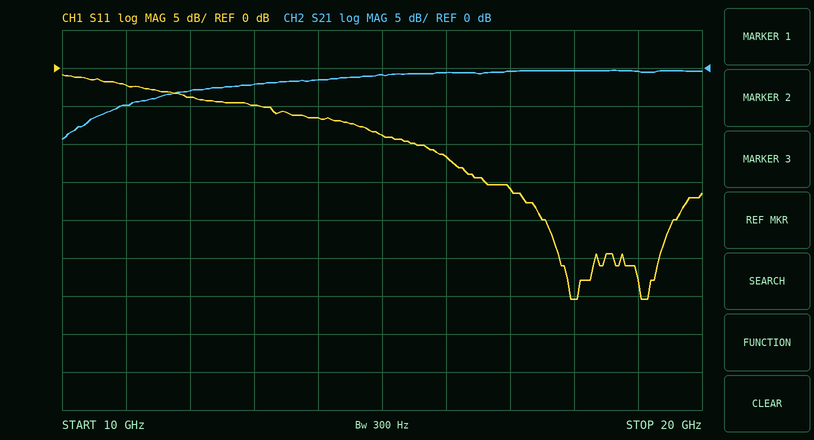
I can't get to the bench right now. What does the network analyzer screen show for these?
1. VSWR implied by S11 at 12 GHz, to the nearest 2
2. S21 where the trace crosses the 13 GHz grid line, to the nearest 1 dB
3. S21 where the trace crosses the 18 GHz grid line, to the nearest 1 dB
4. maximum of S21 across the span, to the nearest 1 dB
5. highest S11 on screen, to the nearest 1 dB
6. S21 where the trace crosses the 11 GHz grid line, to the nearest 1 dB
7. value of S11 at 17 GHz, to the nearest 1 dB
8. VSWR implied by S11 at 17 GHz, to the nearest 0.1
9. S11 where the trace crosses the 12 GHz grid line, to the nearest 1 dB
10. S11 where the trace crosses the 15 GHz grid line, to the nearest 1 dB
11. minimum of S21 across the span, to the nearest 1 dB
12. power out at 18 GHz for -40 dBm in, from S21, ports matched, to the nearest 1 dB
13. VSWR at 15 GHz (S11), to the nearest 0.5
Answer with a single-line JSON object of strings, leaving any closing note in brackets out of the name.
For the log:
{"VSWR implied by S11 at 12 GHz, to the nearest 2": "4", "S21 where the trace crosses the 13 GHz grid line, to the nearest 1 dB": "-2 dB", "S21 where the trace crosses the 18 GHz grid line, to the nearest 1 dB": "0 dB", "maximum of S21 across the span, to the nearest 1 dB": "0 dB", "highest S11 on screen, to the nearest 1 dB": "-1 dB", "S21 where the trace crosses the 11 GHz grid line, to the nearest 1 dB": "-5 dB", "value of S11 at 17 GHz, to the nearest 1 dB": "-16 dB", "VSWR implied by S11 at 17 GHz, to the nearest 0.1": "1.4", "S11 where the trace crosses the 12 GHz grid line, to the nearest 1 dB": "-4 dB", "S11 where the trace crosses the 15 GHz grid line, to the nearest 1 dB": "-9 dB", "minimum of S21 across the span, to the nearest 1 dB": "-9 dB", "power out at 18 GHz for -40 dBm in, from S21, ports matched, to the nearest 1 dB": "-40 dBm", "VSWR at 15 GHz (S11), to the nearest 0.5": "2.0"}
